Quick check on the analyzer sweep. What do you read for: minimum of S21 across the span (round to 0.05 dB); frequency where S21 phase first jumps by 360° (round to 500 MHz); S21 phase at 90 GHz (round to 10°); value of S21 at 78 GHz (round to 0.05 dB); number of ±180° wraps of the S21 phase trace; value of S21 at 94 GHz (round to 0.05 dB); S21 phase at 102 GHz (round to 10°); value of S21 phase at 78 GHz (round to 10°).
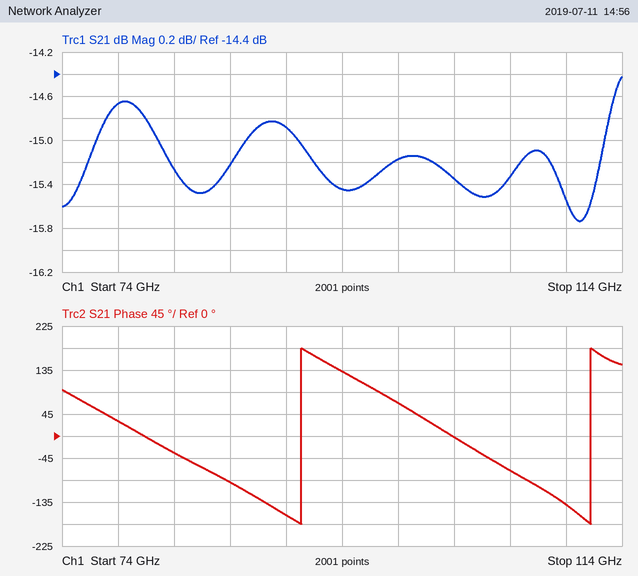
-15.75 dB
91.0 GHz
-160°
-14.65 dB
2
-15.45 dB
0°
30°
